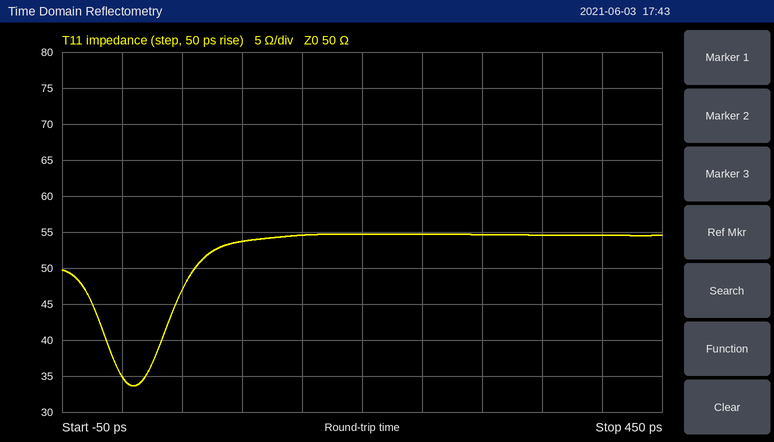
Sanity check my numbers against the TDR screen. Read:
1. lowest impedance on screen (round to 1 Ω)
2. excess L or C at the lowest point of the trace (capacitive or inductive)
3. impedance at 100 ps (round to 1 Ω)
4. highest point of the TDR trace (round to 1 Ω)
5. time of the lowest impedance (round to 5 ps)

34 Ω
capacitive
54 Ω
55 Ω
10 ps
